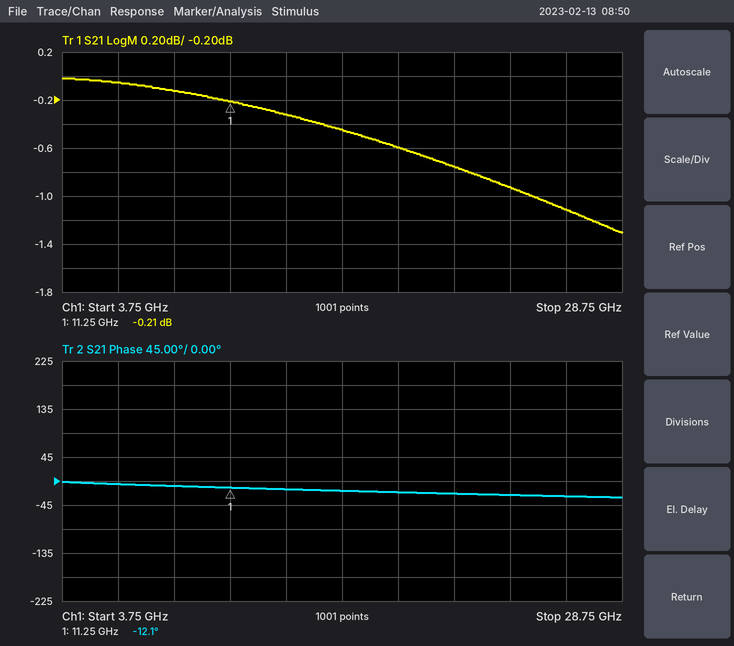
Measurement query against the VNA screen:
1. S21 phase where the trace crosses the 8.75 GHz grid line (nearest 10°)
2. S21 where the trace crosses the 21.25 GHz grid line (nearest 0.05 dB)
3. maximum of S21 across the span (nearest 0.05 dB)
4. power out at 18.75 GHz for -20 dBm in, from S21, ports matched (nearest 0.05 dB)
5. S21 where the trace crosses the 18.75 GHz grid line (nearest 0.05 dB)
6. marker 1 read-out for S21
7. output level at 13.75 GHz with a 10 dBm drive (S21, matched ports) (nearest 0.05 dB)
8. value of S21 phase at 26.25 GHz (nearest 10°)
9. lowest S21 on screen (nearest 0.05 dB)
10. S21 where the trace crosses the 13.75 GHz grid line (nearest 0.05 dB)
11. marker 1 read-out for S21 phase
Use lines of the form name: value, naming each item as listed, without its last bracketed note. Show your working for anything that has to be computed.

S21 phase where the trace crosses the 8.75 GHz grid line: -10°
S21 where the trace crosses the 21.25 GHz grid line: -0.75 dB
maximum of S21 across the span: 0.00 dB
power out at 18.75 GHz for -20 dBm in, from S21, ports matched: -20 dBm + (-0.60 dB) = -20.60 dBm
S21 where the trace crosses the 18.75 GHz grid line: -0.60 dB
marker 1 read-out for S21: -0.21 dB
output level at 13.75 GHz with a 10 dBm drive (S21, matched ports): 10 dBm + (-0.30 dB) = 9.70 dBm
value of S21 phase at 26.25 GHz: -30°
lowest S21 on screen: -1.30 dB
S21 where the trace crosses the 13.75 GHz grid line: -0.30 dB
marker 1 read-out for S21 phase: -12.1°
